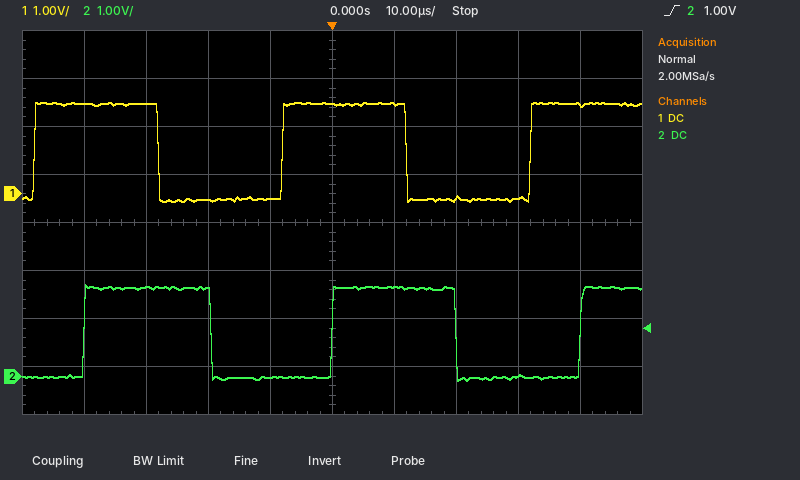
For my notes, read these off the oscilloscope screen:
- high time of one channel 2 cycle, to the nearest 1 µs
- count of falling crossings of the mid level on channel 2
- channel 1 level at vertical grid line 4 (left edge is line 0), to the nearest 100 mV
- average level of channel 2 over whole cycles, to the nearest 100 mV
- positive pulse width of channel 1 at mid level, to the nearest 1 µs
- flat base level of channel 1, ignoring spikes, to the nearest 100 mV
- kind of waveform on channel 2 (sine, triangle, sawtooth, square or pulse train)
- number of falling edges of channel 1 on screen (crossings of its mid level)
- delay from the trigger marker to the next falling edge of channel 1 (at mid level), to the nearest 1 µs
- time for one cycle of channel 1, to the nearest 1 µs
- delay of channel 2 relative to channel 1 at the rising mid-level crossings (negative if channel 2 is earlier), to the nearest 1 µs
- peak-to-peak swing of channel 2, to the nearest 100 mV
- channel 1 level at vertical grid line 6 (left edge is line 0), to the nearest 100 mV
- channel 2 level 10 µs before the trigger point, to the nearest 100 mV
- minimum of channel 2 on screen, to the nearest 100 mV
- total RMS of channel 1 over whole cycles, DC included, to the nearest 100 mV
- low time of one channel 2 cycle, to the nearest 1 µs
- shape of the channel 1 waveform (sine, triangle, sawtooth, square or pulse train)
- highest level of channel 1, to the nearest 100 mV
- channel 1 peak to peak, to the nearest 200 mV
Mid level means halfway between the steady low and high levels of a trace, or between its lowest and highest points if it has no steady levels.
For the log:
20 µs
2
-100 mV
900 mV
20 µs
-100 mV
square
2
12 µs
40 µs
+8 µs
2.0 V
1.9 V
0.0 V
-100 mV
1.3 V
20 µs
square
1.9 V
2.0 V
